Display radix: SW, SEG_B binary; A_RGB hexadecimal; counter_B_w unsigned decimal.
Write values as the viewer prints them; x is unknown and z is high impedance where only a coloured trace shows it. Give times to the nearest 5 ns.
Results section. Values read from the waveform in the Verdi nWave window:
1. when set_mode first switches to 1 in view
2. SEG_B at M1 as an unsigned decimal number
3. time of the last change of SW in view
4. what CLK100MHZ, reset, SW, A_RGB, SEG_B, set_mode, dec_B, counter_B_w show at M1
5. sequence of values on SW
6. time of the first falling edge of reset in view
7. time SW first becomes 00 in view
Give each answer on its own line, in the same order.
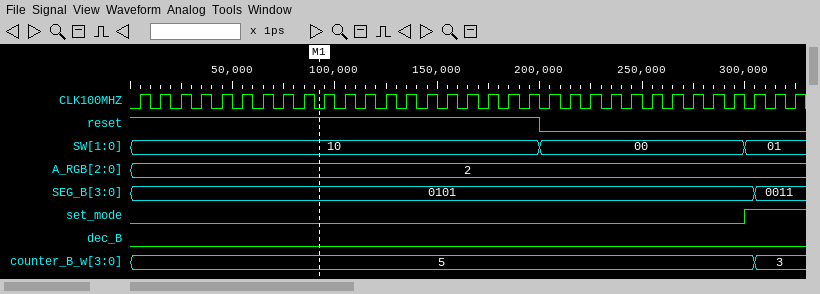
300 ns
5
300 ns
CLK100MHZ=0, reset=1, SW=10, A_RGB=2, SEG_B=0101, set_mode=0, dec_B=0, counter_B_w=5
10, 00, 01
200 ns
200 ns
